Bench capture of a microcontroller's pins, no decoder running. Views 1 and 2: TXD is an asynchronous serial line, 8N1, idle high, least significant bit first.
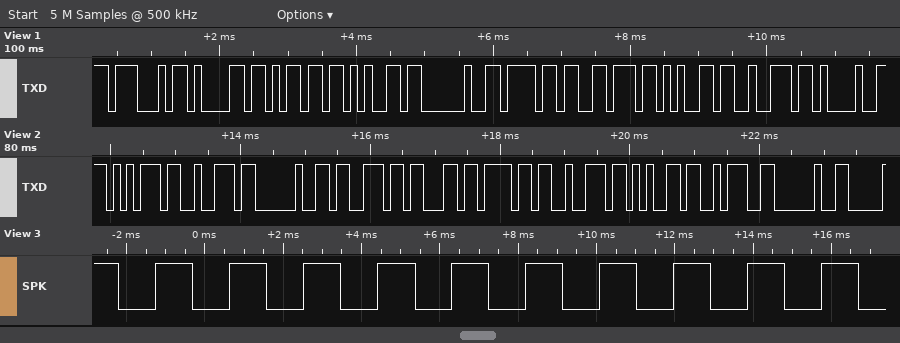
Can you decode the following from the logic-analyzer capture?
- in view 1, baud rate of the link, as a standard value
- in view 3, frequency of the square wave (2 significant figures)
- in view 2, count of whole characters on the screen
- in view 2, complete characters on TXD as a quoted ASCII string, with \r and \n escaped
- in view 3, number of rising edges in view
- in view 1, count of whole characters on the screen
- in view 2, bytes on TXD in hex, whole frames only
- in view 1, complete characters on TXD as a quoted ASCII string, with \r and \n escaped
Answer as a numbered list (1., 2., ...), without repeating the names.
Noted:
1. 9600 baud
2. 530 Hz
3. 10
4. "ur score: "
5. 10
6. 10
7. 75 72 20 73 63 6F 72 65 3A 20
8. "Game over!"
